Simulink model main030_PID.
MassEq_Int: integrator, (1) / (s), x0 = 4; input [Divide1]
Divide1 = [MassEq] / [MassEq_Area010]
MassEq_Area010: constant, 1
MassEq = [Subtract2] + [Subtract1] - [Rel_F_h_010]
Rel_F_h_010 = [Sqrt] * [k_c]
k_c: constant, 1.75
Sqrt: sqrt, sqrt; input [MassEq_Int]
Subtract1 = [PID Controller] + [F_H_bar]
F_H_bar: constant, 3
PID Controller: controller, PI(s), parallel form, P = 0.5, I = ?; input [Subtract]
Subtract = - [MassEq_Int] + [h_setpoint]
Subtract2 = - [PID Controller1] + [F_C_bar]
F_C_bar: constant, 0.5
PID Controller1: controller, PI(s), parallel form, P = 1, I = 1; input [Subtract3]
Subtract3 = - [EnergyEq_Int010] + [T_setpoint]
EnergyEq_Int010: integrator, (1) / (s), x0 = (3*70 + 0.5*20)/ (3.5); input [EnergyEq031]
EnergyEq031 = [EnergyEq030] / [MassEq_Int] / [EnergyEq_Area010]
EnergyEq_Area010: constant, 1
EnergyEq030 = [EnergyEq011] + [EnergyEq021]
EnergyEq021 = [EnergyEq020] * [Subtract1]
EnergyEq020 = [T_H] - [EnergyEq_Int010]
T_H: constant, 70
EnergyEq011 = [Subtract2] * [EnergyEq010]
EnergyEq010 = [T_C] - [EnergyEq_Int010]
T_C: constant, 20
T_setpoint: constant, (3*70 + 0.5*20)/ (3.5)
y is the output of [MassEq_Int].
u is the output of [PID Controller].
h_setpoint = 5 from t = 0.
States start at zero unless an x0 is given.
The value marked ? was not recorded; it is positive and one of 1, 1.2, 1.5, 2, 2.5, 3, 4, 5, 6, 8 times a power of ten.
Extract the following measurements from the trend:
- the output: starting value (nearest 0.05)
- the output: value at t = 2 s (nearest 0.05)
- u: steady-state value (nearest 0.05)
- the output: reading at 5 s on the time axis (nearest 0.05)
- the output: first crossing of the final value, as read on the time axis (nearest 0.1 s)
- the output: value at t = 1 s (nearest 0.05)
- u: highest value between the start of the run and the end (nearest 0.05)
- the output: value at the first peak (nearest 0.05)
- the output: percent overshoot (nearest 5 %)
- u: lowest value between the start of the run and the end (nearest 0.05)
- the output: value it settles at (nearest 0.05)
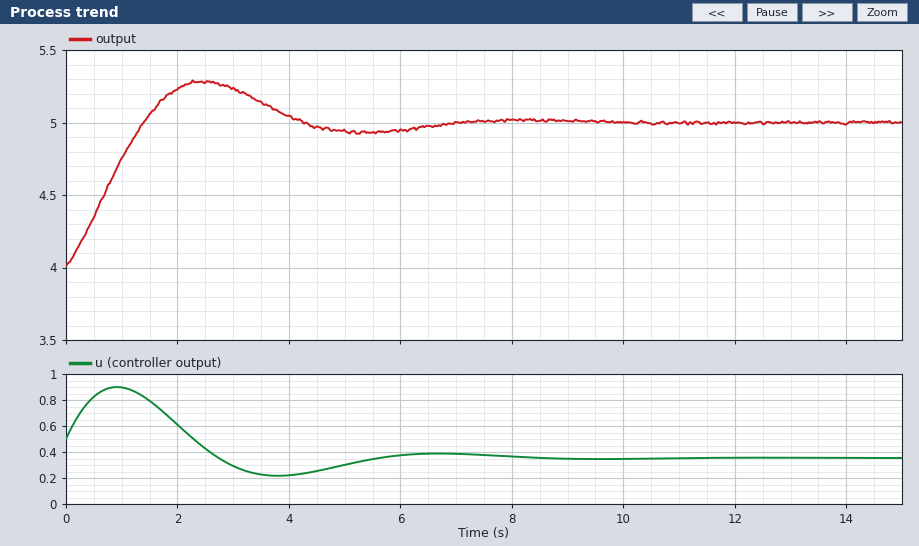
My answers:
4.00
5.25
0.35
4.95
1.4 s
4.75
0.90
5.30
30 %
0.20
5.00
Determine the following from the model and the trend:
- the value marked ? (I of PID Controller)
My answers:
1.2
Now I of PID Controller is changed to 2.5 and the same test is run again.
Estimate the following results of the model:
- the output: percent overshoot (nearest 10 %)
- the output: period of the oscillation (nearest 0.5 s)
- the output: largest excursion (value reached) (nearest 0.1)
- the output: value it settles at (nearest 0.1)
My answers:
40 %
4.0 s
5.4
5.0
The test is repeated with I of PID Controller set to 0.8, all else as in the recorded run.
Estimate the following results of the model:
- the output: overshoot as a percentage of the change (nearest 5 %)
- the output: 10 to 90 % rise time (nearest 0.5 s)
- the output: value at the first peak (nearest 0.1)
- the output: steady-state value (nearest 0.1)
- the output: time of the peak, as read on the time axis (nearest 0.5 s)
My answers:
20 %
1.5 s
5.2
5.0
3.0 s
